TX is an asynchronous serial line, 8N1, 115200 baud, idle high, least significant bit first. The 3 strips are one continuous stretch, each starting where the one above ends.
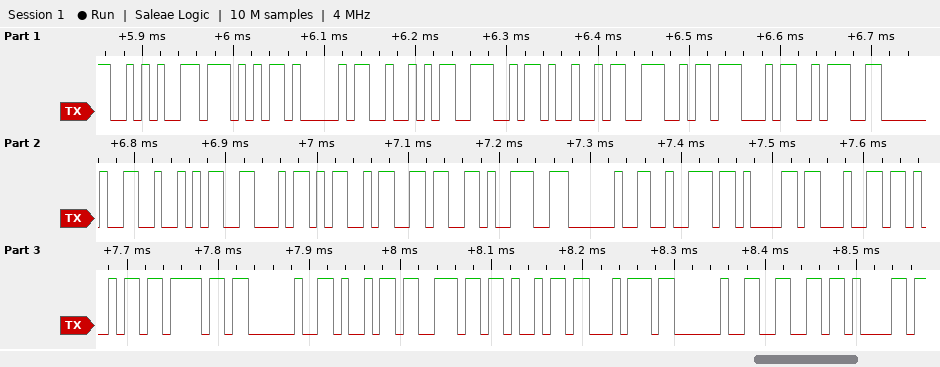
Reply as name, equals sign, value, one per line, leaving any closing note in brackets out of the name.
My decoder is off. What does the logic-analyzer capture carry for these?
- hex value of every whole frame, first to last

hex value of every whole frame, first to last = 0x2A 0x57 0x41 0x52 0x4E 0x49 0x4E 0x47 0x3A 0x20 0x52 0x46 0x4D 0x36 0x39 0x20 0x72 0x61 0x64 0x69 0x6F 0x20 0x69 0x6E 0x69 0x74 0x20 0x66 0x61
